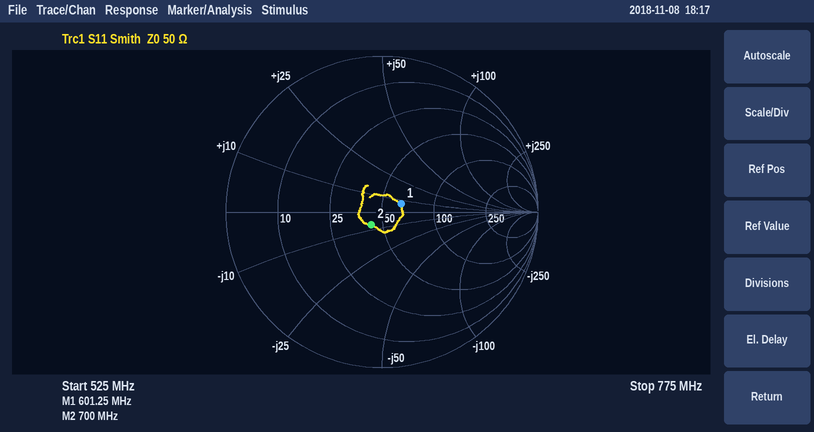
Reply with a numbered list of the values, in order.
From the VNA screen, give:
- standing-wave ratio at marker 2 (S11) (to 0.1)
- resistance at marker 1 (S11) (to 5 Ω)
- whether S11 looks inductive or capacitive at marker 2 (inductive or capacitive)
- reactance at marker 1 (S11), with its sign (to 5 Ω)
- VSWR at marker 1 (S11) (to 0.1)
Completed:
1. 1.2
2. 65 Ω
3. capacitive
4. +5 Ω
5. 1.3
